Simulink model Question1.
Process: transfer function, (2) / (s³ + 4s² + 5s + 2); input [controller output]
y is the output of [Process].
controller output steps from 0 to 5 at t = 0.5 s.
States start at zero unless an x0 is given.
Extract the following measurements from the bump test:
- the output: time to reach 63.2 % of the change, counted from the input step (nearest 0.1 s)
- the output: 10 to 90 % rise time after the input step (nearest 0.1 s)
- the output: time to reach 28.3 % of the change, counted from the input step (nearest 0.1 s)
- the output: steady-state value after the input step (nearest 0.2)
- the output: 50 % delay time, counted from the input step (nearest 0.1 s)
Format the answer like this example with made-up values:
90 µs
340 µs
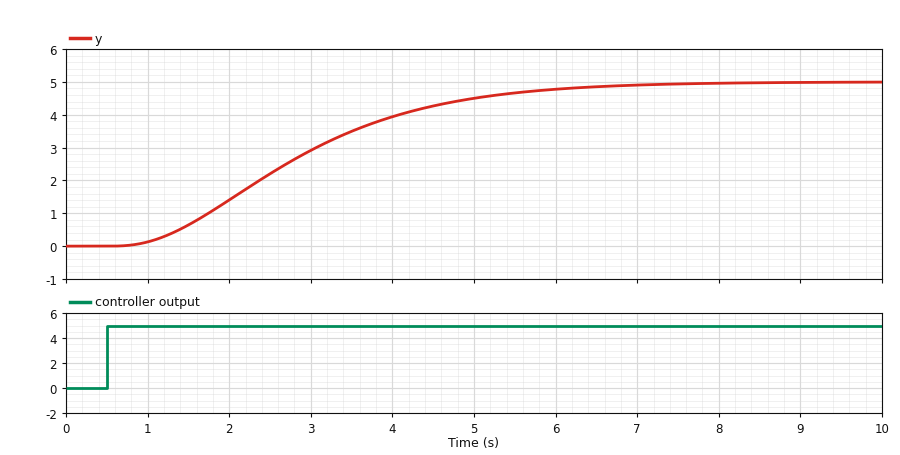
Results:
2.7 s
3.6 s
1.5 s
5.0
2.2 s
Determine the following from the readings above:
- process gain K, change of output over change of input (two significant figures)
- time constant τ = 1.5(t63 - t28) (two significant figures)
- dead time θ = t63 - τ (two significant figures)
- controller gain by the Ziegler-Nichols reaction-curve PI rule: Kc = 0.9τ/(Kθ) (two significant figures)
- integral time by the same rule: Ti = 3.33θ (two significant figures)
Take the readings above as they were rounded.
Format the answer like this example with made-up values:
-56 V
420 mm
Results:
1.0
1.8 s
0.90 s
1.8
3.0 s
